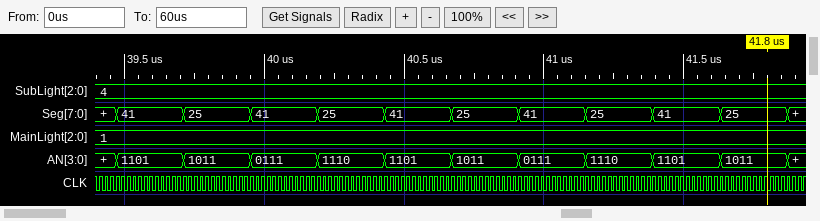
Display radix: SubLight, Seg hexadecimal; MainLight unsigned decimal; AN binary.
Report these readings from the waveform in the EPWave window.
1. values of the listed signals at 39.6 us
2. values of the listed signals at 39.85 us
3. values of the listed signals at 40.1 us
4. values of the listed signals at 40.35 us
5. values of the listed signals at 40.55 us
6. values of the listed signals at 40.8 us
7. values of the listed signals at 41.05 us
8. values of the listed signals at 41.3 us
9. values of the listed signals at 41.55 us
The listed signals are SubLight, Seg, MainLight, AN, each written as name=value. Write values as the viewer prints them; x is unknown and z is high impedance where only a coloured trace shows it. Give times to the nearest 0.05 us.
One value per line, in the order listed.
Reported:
SubLight=4, Seg=41, MainLight=1, AN=1101
SubLight=4, Seg=25, MainLight=1, AN=1011
SubLight=4, Seg=41, MainLight=1, AN=0111
SubLight=4, Seg=25, MainLight=1, AN=1110
SubLight=4, Seg=41, MainLight=1, AN=1101
SubLight=4, Seg=25, MainLight=1, AN=1011
SubLight=4, Seg=41, MainLight=1, AN=0111
SubLight=4, Seg=25, MainLight=1, AN=1110
SubLight=4, Seg=41, MainLight=1, AN=1101
